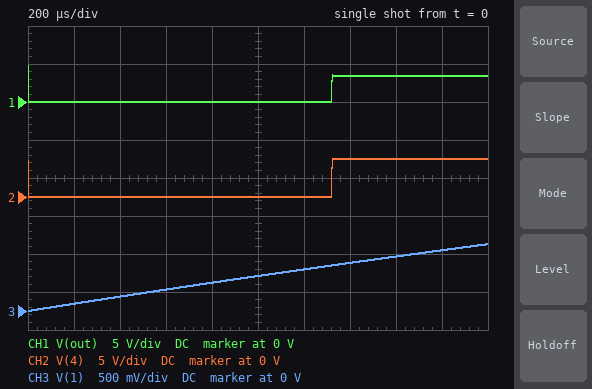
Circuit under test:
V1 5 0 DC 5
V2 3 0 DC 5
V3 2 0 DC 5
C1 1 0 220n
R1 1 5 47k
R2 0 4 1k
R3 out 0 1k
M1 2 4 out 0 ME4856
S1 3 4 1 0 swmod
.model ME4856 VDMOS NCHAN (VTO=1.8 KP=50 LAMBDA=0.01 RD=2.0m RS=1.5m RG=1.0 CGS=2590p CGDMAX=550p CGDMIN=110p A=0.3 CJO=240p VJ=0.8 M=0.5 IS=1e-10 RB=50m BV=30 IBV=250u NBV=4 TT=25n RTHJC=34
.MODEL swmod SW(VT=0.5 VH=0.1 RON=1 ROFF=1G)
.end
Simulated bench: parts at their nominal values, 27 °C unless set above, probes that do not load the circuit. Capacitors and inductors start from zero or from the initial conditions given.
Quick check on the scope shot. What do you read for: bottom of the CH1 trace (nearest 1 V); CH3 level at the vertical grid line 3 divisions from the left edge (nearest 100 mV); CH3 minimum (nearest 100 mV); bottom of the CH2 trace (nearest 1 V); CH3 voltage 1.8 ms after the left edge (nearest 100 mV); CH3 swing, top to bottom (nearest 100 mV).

0 V
300 mV
0 V
0 V
800 mV
900 mV
